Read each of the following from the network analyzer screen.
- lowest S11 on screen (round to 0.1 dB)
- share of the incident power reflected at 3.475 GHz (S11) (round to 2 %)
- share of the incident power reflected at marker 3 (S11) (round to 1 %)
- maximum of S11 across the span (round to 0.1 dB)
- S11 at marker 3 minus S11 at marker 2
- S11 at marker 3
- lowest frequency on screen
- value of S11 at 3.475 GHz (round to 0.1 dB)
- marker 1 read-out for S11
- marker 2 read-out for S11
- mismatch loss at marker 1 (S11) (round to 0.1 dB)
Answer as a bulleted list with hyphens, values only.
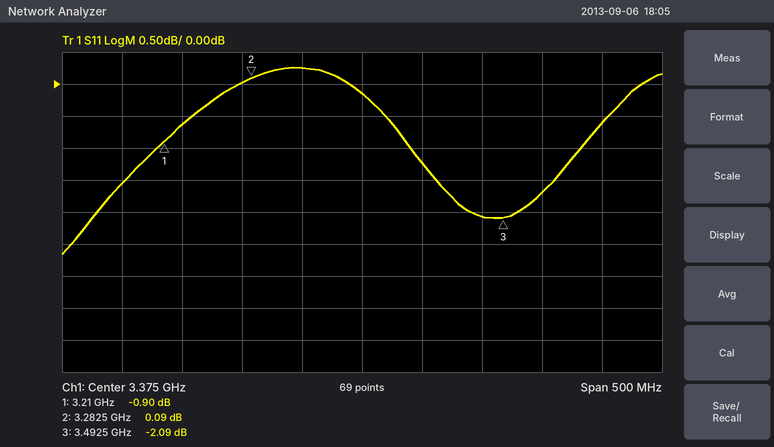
- -2.7 dB
- 62 %
- 62 %
- 0.3 dB
- -2.18 dB
- -2.09 dB
- 3.125 GHz
- -2.1 dB
- -0.90 dB
- 0.09 dB
- 7.3 dB
